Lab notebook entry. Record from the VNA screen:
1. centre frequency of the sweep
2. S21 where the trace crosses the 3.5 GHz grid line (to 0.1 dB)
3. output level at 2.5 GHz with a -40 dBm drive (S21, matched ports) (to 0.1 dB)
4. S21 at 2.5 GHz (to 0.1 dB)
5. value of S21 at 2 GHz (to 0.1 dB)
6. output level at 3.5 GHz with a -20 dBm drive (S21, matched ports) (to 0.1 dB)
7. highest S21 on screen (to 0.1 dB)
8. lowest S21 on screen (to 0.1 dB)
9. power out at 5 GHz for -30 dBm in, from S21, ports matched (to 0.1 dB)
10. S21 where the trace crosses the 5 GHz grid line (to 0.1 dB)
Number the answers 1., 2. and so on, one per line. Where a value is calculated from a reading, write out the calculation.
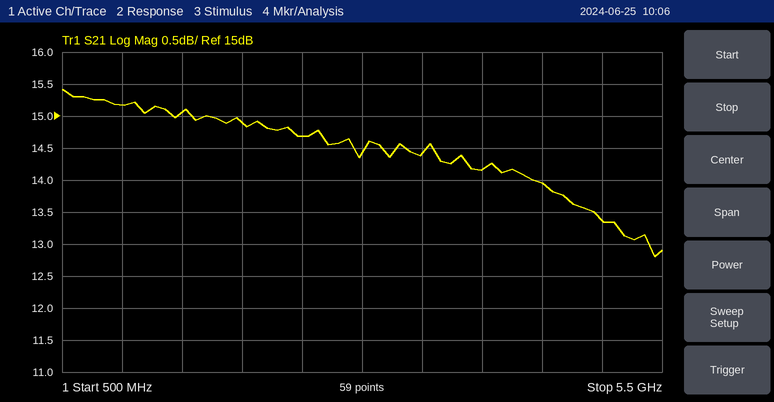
1. 3 GHz
2. 14.4 dB
3. -40 dBm + (14.7 dB) = -25.3 dBm
4. 14.7 dB
5. 14.9 dB
6. -20 dBm + (14.4 dB) = -5.6 dBm
7. 15.4 dB
8. 12.8 dB
9. -30 dBm + (13.4 dB) = -16.6 dBm
10. 13.4 dB
